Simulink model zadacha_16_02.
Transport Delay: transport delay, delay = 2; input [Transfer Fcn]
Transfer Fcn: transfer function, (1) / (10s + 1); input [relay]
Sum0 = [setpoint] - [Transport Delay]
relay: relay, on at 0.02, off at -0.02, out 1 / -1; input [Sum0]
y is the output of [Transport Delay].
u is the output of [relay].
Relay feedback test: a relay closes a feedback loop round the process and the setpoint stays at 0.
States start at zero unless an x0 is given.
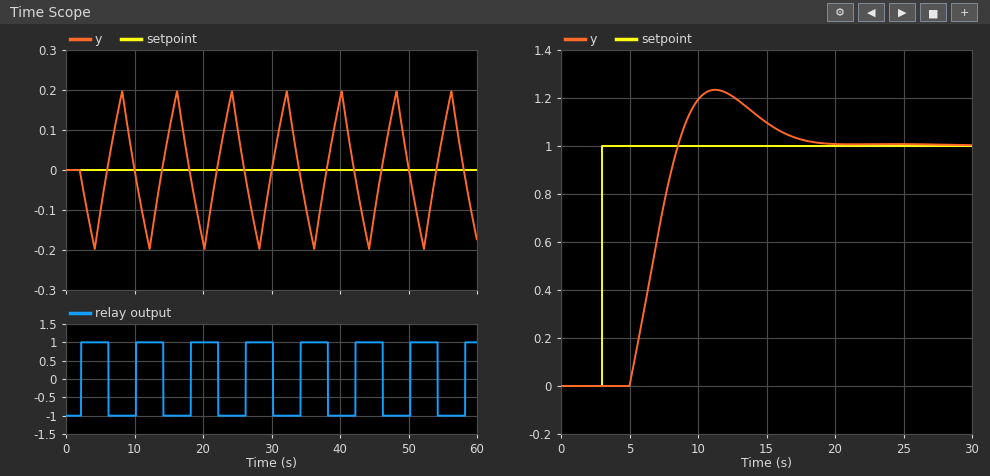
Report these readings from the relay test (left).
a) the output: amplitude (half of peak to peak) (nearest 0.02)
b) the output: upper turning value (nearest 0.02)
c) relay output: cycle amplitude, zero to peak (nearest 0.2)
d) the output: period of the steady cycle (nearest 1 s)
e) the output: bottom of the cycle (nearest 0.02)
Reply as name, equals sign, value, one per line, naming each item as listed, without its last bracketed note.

the output: amplitude (half of peak to peak) = 0.20
the output: upper turning value = 0.20
relay output: cycle amplitude, zero to peak = 1.0
the output: period of the steady cycle = 8 s
the output: bottom of the cycle = -0.20
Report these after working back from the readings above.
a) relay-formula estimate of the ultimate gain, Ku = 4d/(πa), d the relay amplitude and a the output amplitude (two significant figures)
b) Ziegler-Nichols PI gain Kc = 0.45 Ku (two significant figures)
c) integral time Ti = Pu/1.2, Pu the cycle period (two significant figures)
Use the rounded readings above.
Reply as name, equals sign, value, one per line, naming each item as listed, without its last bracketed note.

relay-formula estimate of the ultimate gain, Ku = 4d/(πa), d the relay amplitude and a the output amplitude = 6.4
Ziegler-Nichols PI gain Kc = 0.45 Ku = 2.9
integral time Ti = Pu/1.2, Pu the cycle period = 6.7 s
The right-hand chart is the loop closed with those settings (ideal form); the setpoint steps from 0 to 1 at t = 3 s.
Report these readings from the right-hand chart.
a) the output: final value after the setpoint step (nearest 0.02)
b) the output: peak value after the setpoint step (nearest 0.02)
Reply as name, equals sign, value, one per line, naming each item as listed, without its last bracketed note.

the output: final value after the setpoint step = 1.00
the output: peak value after the setpoint step = 1.24
